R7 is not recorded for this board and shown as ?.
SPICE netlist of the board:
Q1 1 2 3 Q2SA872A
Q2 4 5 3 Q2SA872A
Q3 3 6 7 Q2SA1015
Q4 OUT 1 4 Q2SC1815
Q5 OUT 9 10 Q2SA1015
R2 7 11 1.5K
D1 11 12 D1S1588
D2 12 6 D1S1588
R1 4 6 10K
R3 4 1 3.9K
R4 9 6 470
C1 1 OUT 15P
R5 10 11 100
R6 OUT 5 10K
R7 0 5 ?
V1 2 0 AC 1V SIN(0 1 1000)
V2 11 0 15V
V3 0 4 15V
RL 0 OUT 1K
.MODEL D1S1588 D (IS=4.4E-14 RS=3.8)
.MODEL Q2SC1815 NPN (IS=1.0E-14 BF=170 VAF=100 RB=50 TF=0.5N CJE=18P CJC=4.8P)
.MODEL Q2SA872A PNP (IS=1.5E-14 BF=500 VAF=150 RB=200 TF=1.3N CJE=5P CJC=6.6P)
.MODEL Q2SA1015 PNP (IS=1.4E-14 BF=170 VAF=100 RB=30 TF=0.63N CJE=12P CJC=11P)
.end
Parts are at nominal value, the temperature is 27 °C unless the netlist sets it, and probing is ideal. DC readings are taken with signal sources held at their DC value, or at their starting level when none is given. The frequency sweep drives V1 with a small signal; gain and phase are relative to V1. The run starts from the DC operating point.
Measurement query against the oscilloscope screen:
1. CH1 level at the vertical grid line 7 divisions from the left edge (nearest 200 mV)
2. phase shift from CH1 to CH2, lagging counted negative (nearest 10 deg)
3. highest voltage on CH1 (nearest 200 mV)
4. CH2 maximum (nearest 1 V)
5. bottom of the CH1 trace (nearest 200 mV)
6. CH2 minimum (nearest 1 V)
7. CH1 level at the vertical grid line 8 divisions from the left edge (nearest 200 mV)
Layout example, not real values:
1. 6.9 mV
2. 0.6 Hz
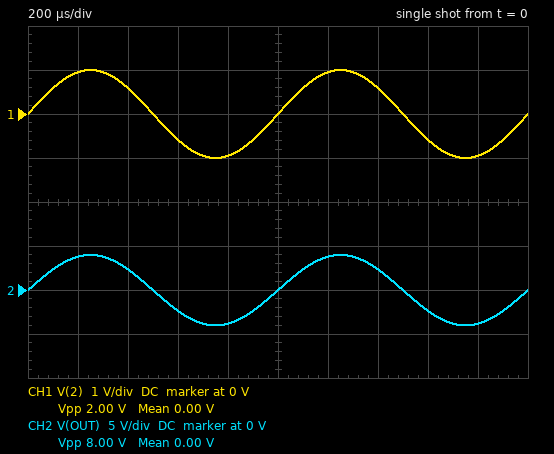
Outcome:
1. 600 mV
2. 0 deg
3. 1.0 V
4. 4 V
5. -1.0 V
6. -4 V
7. -600 mV
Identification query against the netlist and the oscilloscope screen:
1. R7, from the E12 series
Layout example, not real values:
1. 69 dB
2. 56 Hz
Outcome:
1. 3.3 kΩ
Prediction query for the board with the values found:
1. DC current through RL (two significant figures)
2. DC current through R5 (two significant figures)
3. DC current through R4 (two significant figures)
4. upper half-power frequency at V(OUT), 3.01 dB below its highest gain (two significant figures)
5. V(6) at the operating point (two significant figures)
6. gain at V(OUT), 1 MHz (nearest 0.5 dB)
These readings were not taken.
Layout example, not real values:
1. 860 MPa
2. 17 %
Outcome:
1. 19 µA
2. 6.0 mA
3. 31 µA
4. 8.1 MHz
5. 14 V
6. 12.0 dB
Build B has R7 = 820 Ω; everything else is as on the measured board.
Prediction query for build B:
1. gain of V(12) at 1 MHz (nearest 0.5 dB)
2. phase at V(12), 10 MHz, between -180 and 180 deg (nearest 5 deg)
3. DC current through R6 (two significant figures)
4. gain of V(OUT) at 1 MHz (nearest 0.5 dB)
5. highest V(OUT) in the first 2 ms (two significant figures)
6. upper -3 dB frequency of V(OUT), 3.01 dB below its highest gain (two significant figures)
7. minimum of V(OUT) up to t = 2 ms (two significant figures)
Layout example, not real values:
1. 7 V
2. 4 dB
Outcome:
1. -47.0 dB
2. -45 deg
3. 4.9 µA
4. 22.0 dB
5. 5.5 V
6. 4.0 MHz
7. -13 V
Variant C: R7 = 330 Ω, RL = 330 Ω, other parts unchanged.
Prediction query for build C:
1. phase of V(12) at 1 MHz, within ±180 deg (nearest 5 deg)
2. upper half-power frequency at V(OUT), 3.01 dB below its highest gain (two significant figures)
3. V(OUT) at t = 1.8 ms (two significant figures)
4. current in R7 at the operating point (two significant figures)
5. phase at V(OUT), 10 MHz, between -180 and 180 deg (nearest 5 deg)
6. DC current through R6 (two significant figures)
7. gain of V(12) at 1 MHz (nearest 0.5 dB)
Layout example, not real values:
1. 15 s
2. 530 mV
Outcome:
1. 50 deg
2. 1.4 MHz
3. -12 V
4. 9.8 µA
5. -115 deg
6. 10 µA
7. -42.5 dB
